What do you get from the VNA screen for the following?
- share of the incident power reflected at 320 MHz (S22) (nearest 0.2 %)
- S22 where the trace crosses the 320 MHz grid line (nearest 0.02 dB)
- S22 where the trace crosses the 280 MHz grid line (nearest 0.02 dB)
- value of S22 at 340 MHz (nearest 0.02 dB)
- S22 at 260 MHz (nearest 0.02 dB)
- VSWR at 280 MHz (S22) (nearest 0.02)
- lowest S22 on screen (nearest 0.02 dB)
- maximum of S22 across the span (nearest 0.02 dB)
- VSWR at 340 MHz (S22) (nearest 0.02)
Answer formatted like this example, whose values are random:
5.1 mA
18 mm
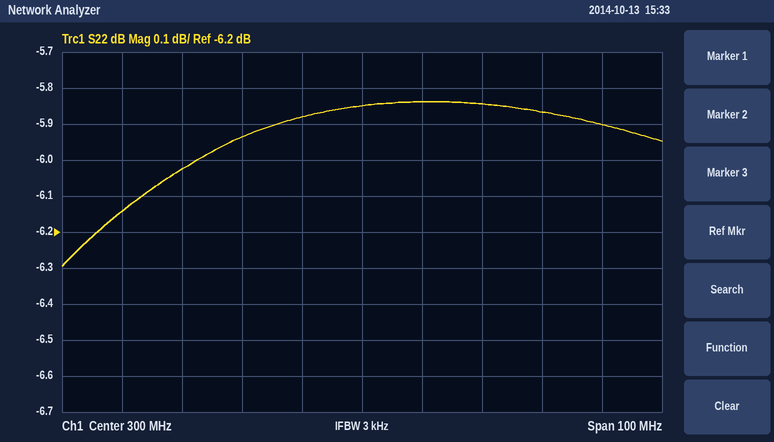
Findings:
26.0 %
-5.84 dB
-5.94 dB
-5.90 dB
-6.14 dB
3.04
-6.30 dB
-5.84 dB
3.06
